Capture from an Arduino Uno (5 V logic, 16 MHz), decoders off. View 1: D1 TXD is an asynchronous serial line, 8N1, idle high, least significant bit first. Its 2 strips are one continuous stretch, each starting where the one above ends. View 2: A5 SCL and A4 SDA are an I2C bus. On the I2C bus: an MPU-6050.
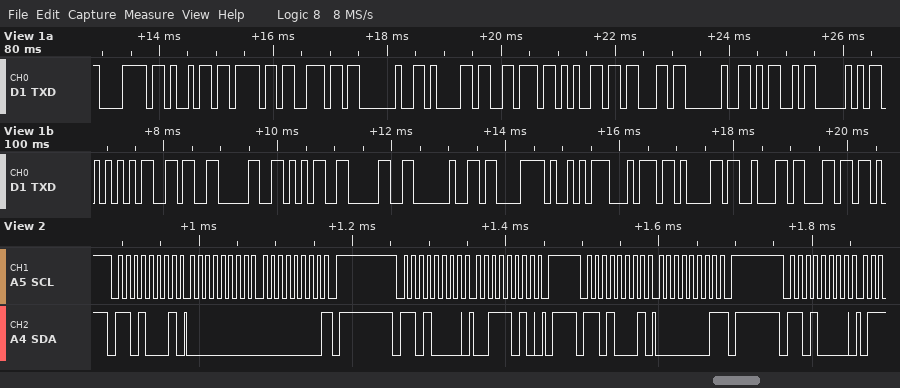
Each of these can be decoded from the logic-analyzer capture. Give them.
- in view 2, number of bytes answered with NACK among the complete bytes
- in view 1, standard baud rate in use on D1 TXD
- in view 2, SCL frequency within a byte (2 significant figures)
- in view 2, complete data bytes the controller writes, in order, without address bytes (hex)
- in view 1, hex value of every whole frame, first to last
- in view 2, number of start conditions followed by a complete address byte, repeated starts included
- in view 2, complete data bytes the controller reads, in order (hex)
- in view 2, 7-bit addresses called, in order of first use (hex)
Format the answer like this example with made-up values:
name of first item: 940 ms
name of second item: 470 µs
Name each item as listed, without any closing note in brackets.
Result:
in view 2, number of bytes answered with NACK among the complete bytes: 2
in view 1, standard baud rate in use on D1 TXD: 9600 baud
in view 2, SCL frequency within a byte: 100 kHz
in view 2, complete data bytes the controller writes, in order, without address bytes: 3A
in view 1, hex value of every whole frame, first to last: 78 69 6F 6E 20 61 76 65 63 20 4D 50 55 36 30 35 30 20 C3 A9 74 61 62 6C
in view 2, number of start conditions followed by a complete address byte, repeated starts included: 4
in view 2, complete data bytes the controller reads, in order: 00 00 01
in view 2, 7-bit addresses called, in order of first use: 0x68
